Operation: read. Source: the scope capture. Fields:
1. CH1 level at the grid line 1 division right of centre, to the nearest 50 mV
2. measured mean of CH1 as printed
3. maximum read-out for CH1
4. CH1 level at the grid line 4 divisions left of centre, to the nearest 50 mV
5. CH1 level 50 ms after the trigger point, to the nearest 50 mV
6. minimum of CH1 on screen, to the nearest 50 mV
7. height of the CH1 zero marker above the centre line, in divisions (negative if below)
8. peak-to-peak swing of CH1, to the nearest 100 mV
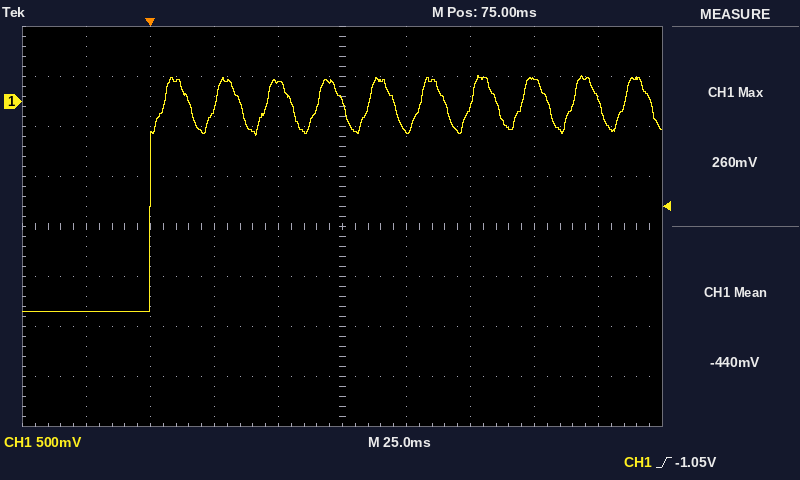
-300 mV
-440 mV
260 mV
-2.10 V
200 mV
-2.10 V
+2.5 div
2.40 V
